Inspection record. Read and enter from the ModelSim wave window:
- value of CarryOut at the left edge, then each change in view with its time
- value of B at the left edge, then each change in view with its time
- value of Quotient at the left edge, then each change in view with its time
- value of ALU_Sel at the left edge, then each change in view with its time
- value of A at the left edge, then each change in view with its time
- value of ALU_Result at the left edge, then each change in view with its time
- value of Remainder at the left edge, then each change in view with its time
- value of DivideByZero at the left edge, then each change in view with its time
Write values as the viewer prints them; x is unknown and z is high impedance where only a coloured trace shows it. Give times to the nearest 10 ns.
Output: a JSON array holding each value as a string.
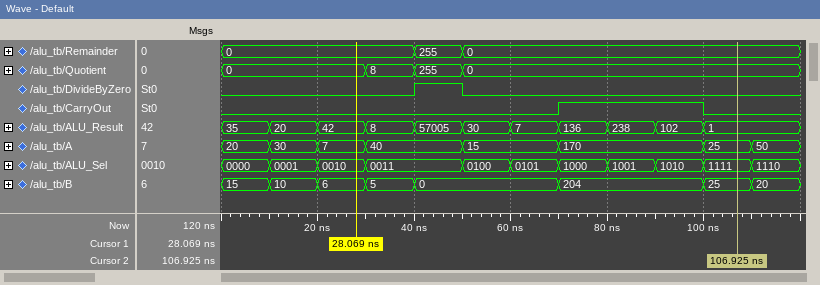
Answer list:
["0, 1 at 70 ns, 0 at 100 ns", "15, 10 at 10 ns, 6 at 20 ns, 5 at 30 ns, 0 at 40 ns, 204 at 70 ns, 25 at 100 ns, 20 at 110 ns", "0, 8 at 30 ns, 255 at 40 ns, 0 at 50 ns", "0000, 0001 at 10 ns, 0010 at 20 ns, 0011 at 30 ns, 0100 at 50 ns, 0101 at 60 ns, 1000 at 70 ns, 1001 at 80 ns, 1010 at 90 ns, 1111 at 100 ns, 1110 at 110 ns", "20, 30 at 10 ns, 7 at 20 ns, 40 at 30 ns, 15 at 50 ns, 170 at 70 ns, 25 at 100 ns, 50 at 110 ns", "35, 20 at 10 ns, 42 at 20 ns, 8 at 30 ns, 57005 at 40 ns, 30 at 50 ns, 7 at 60 ns, 136 at 70 ns, 238 at 80 ns, 102 at 90 ns, 1 at 100 ns", "0, 255 at 40 ns, 0 at 50 ns", "0, 1 at 40 ns, 0 at 50 ns"]
